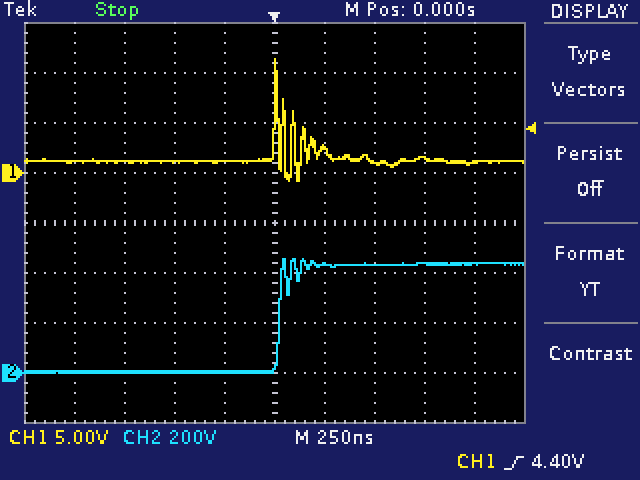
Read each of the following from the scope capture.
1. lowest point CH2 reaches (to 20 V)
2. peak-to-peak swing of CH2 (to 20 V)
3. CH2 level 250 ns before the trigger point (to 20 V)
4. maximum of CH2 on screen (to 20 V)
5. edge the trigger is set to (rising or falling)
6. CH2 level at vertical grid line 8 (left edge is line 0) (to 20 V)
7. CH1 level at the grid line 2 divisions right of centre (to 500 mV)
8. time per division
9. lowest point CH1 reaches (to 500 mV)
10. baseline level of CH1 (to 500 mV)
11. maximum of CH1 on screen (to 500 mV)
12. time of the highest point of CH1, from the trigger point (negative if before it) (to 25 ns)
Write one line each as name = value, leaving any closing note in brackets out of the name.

lowest point CH2 reaches = 0 V
peak-to-peak swing of CH2 = 460 V
CH2 level 250 ns before the trigger point = 0 V
maximum of CH2 on screen = 460 V
edge the trigger is set to = rising
CH2 level at vertical grid line 8 (left edge is line 0) = 440 V
CH1 level at the grid line 2 divisions right of centre = 1.0 V
time per division = 250 ns
lowest point CH1 reaches = -1.0 V
baseline level of CH1 = 1.0 V
maximum of CH1 on screen = 11.5 V
time of the highest point of CH1, from the trigger point (negative if before it) = 0 ns
